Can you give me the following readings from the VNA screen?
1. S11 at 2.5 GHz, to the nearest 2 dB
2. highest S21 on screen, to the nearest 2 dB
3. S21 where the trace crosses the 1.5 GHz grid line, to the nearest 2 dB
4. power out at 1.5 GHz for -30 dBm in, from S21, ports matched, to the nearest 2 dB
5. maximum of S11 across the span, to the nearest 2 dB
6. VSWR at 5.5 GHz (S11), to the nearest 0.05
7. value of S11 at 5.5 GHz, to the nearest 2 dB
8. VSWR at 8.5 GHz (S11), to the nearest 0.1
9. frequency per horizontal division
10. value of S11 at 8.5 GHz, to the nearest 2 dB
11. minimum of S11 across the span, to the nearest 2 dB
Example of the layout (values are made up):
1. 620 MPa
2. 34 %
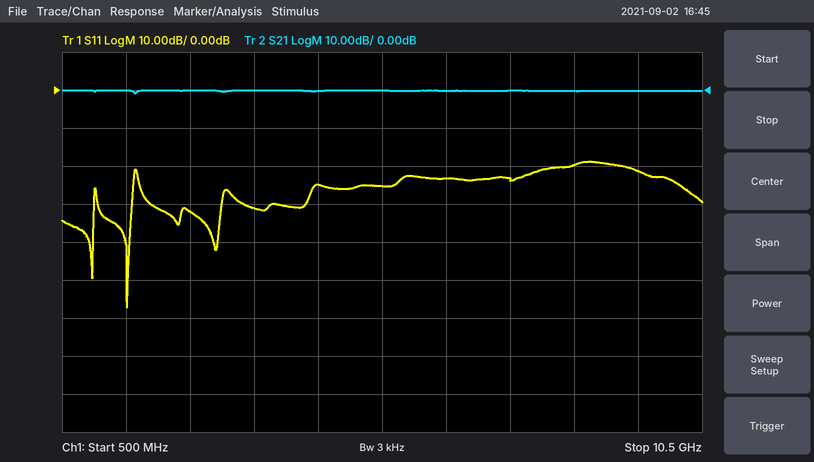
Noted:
1. -32 dB
2. 0 dB
3. 0 dB
4. -30 dBm
5. -18 dB
6. 1.10
7. -26 dB
8. 1.2
9. 1 GHz
10. -20 dB
11. -58 dB
